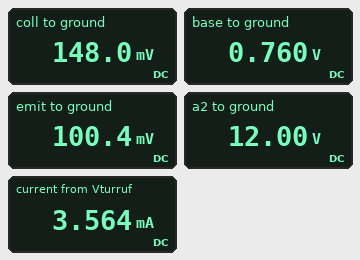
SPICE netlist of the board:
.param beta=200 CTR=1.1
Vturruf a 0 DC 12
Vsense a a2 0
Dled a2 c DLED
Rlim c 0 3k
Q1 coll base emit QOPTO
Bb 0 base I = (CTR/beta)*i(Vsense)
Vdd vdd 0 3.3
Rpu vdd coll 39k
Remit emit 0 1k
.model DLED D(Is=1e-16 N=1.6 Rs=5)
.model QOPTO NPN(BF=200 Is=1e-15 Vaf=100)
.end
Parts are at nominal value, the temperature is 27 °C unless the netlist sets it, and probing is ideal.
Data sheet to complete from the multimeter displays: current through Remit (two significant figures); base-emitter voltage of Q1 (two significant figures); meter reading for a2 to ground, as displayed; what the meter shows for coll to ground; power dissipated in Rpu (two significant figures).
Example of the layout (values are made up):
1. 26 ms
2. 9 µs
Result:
1. 100 µA
2. 660 mV
3. 12.00 V
4. 148.0 mV
5. 250 µW
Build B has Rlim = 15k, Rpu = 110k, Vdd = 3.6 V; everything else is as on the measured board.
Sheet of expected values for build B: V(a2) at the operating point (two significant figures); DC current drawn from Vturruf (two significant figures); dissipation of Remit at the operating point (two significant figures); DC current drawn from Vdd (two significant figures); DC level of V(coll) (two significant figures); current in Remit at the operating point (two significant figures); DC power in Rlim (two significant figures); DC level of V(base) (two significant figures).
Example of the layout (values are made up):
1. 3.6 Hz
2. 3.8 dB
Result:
1. 12 V
2. 720 µA
3. 1.3 µW
4. 32 µA
5. 97 mV
6. 36 µA
7. 7.7 mW
8. 670 mV
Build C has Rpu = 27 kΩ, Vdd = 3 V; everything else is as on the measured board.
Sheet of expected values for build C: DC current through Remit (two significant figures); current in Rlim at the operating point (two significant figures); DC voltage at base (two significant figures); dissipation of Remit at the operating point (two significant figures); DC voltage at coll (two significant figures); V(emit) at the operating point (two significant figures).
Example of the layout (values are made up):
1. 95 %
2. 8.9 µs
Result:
1. 120 µA
2. 3.6 mA
3. 790 mV
4. 15 µW
5. 180 mV
6. 120 mV
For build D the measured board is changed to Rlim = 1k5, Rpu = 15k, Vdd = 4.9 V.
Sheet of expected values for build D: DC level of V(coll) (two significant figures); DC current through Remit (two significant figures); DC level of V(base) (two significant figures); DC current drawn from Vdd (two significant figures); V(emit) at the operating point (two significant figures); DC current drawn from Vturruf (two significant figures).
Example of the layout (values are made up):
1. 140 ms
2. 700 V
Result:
1. 400 mV
2. 340 µA
3. 1.0 V
4. 300 µA
5. 340 mV
6. 7.1 mA
